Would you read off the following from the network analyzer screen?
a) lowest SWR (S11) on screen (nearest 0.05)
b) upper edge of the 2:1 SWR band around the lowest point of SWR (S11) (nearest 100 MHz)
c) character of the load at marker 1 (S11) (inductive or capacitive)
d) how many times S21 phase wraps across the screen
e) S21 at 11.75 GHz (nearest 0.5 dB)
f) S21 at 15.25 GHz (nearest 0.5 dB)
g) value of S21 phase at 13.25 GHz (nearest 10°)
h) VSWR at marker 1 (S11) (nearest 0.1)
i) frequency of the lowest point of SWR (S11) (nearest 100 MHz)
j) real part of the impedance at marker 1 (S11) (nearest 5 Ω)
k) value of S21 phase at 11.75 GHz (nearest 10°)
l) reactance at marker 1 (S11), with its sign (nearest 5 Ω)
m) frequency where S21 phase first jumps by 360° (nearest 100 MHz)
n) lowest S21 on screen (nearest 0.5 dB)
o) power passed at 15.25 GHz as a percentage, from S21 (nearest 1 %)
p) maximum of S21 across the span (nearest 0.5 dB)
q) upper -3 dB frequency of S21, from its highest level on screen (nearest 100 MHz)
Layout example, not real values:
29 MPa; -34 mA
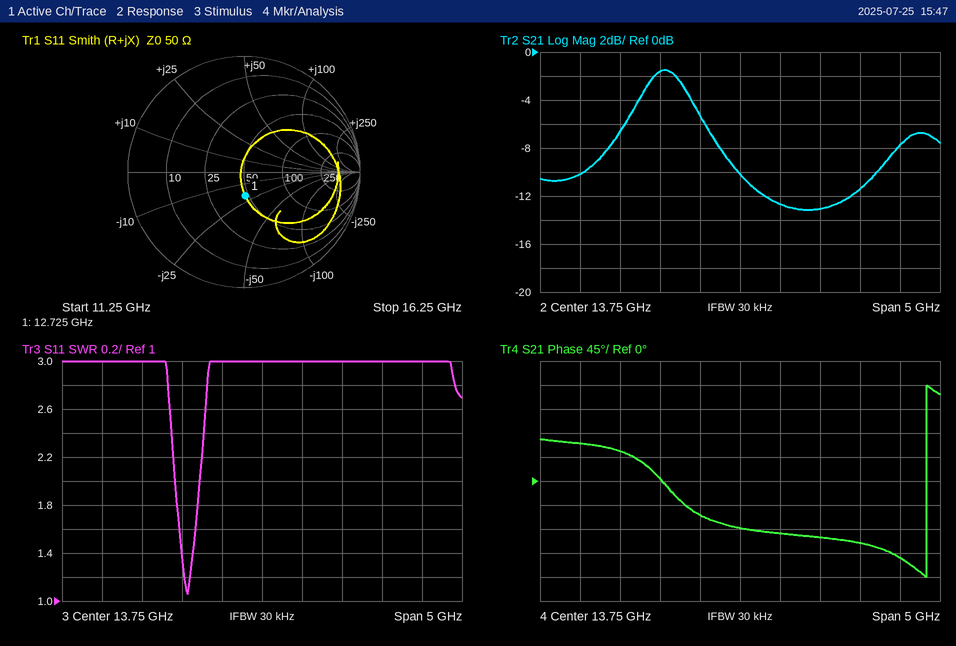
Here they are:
1.05; 13.0 GHz; capacitive; 1; -10.0 dB; -11.5 dB; -60°; 1.5; 12.8 GHz; 45 Ω; 70°; -20 Ω; 16.1 GHz; -13.0 dB; 7 %; -1.5 dB; 13.2 GHz
